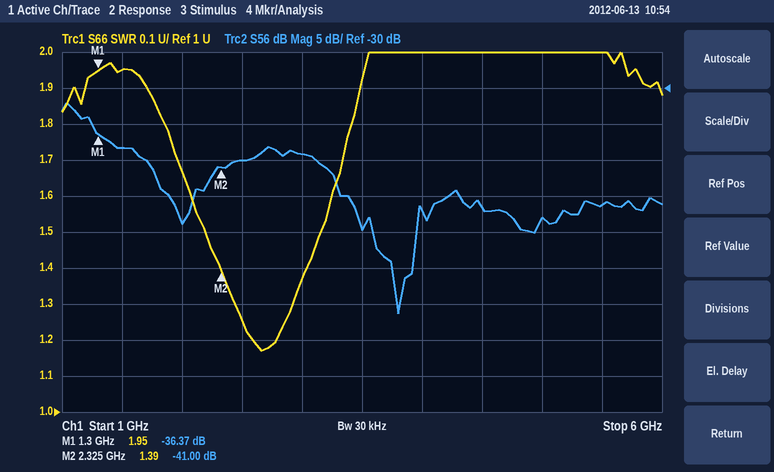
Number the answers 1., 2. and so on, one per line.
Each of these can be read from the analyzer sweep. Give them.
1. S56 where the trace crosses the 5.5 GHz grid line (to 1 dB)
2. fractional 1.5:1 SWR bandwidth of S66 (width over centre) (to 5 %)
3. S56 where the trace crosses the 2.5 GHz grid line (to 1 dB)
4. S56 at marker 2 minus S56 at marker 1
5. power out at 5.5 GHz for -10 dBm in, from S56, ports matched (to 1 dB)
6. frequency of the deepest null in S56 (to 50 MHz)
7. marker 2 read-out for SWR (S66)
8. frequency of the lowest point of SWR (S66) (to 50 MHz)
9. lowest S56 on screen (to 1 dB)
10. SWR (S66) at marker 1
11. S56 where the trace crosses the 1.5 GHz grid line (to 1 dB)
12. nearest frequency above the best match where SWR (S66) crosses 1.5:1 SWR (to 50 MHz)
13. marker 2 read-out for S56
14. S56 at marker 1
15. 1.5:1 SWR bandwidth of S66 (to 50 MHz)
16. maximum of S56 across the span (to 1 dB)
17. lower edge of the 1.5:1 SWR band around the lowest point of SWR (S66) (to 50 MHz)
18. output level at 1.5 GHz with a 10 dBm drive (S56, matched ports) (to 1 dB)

1. -46 dB
2. 35 %
3. -40 dB
4. -4.63 dB
5. -56 dBm
6. 3.80 GHz
7. 1.39
8. 2.65 GHz
9. -61 dB
10. 1.95
11. -38 dB
12. 3.15 GHz
13. -41.00 dB
14. -36.37 dB
15. 950 MHz
16. -32 dB
17. 2.20 GHz
18. -28 dBm
